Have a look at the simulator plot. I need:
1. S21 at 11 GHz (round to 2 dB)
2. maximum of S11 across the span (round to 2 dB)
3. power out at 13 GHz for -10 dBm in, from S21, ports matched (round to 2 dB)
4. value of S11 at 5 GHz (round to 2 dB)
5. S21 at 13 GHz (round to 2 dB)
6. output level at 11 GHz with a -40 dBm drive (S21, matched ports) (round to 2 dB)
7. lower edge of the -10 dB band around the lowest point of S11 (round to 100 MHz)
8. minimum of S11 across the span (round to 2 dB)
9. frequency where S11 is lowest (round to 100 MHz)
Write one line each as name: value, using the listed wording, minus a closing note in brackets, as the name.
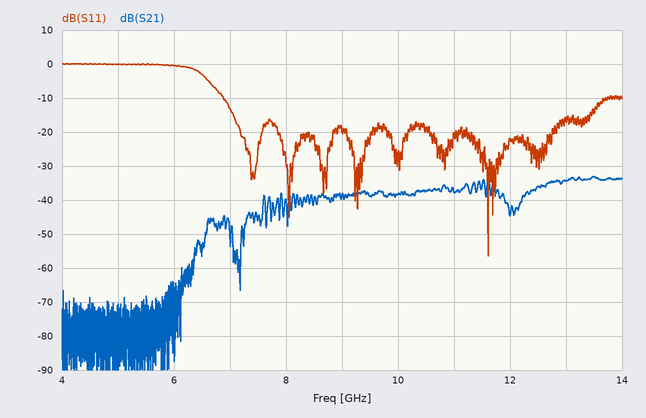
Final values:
S21 at 11 GHz: -38 dB
maximum of S11 across the span: 0 dB
power out at 13 GHz for -10 dBm in, from S21, ports matched: -44 dBm
value of S11 at 5 GHz: 0 dB
S21 at 13 GHz: -34 dB
output level at 11 GHz with a -40 dBm drive (S21, matched ports): -78 dBm
lower edge of the -10 dB band around the lowest point of S11: 6.9 GHz
minimum of S11 across the span: -56 dB
frequency where S11 is lowest: 11.6 GHz
